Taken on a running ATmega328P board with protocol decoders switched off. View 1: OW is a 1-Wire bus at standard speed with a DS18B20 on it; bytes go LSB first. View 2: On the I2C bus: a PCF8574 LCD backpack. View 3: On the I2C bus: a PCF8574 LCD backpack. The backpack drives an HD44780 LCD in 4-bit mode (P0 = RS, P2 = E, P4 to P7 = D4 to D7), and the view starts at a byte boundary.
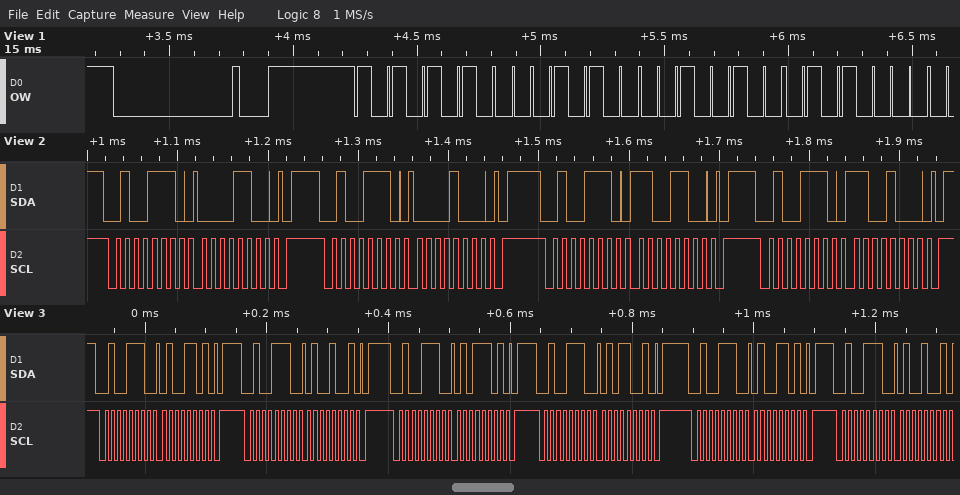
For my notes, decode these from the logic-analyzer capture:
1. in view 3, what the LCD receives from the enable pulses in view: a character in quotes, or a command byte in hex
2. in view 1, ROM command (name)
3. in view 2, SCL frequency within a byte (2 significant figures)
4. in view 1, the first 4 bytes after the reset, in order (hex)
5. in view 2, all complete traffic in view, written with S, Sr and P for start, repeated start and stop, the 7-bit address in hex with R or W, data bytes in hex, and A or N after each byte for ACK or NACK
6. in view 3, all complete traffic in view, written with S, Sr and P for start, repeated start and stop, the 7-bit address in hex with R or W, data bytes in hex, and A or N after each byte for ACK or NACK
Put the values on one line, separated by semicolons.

'E'; Match ROM; 100 kHz; 55 28 24 0A; S 27W A 0C A P S 27W A 08 A P S 27W A CC A P S 27W A C8 A P; S 27W A 4D A P S 27W A 49 A P S 27W A 5D A P S 27W A 59 A P S 27W A 4D A P S 27W A 49 A
